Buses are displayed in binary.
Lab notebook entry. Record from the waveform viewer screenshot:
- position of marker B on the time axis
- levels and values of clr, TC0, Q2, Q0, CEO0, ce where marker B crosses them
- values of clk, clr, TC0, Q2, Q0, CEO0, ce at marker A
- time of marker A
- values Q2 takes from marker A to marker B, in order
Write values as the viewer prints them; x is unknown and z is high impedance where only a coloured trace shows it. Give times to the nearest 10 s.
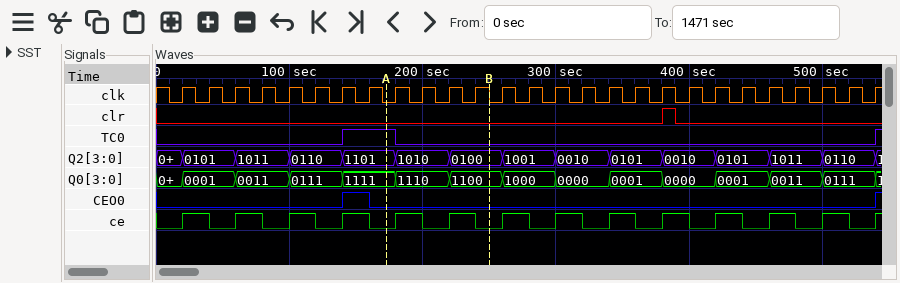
250 s
clr=0, TC0=0, Q2=0100, Q0=1100, CEO0=0, ce=0
clk=0, clr=0, TC0=1, Q2=1101, Q0=1111, CEO0=0, ce=0
170 s
1101, 1010, 0100
